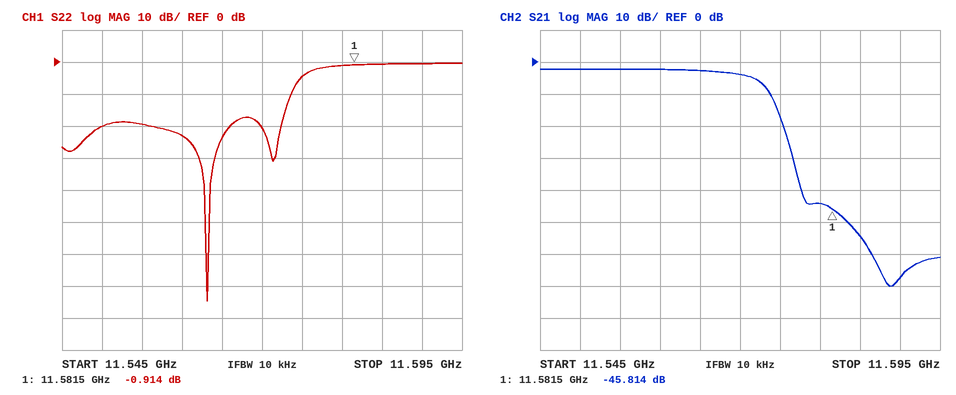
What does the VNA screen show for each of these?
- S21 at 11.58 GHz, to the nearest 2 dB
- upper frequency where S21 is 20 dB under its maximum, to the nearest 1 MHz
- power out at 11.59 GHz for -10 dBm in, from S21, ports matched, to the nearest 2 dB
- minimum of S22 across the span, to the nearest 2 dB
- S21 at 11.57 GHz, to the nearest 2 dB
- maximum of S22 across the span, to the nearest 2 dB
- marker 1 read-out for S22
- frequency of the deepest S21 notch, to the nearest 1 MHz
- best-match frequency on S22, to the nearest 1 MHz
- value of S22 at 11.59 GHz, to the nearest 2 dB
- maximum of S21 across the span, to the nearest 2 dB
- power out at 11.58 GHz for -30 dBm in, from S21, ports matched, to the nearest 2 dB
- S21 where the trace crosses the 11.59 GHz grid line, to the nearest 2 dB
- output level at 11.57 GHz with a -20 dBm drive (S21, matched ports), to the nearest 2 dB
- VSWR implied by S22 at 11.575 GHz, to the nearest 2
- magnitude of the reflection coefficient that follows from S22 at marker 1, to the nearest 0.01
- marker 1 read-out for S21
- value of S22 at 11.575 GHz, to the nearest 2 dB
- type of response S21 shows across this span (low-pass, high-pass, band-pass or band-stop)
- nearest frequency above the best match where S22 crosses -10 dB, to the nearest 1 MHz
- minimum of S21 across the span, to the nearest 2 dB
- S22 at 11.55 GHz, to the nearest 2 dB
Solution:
-44 dB
11.576 GHz
-78 dBm
-74 dB
-4 dB
0 dB
-0.914 dB
11.589 GHz
11.563 GHz
0 dB
-2 dB
-74 dBm
-68 dB
-24 dBm
4
0.90
-45.814 dB
-4 dB
low-pass
11.574 GHz
-70 dB
-20 dB
